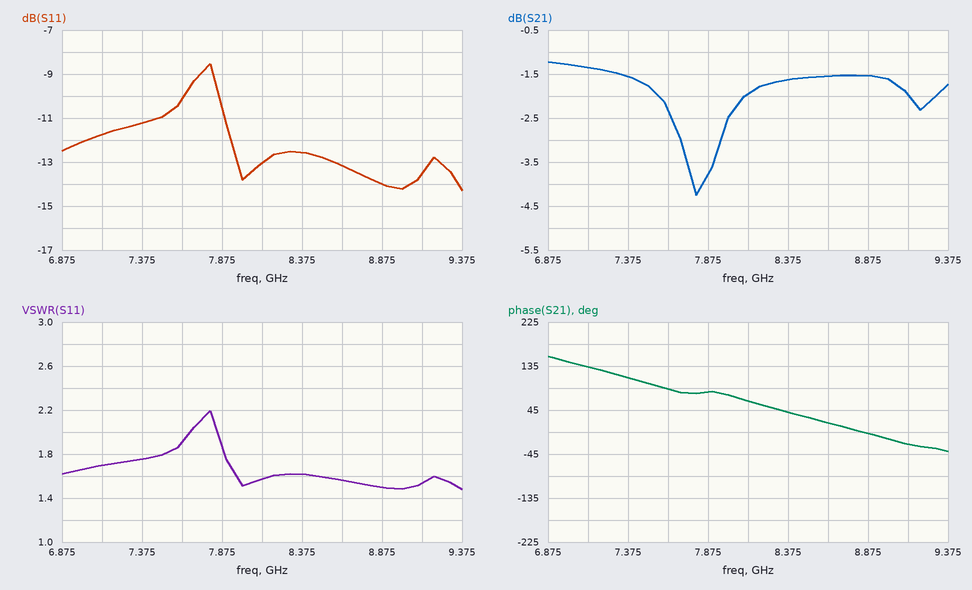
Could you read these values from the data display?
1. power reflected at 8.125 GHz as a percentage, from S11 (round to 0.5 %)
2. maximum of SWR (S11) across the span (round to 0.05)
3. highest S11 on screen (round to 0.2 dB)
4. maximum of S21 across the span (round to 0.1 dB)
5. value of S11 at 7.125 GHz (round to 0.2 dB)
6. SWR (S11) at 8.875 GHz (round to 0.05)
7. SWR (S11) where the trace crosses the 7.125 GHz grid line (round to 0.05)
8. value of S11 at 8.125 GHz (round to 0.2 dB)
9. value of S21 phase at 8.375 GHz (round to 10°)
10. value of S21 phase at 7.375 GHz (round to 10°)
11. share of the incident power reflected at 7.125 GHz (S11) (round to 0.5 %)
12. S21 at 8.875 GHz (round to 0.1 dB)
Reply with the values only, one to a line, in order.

5.0 %
2.20
-8.6 dB
-1.2 dB
-11.8 dB
1.50
1.70
-13.0 dB
40°
110°
6.5 %
-1.5 dB
